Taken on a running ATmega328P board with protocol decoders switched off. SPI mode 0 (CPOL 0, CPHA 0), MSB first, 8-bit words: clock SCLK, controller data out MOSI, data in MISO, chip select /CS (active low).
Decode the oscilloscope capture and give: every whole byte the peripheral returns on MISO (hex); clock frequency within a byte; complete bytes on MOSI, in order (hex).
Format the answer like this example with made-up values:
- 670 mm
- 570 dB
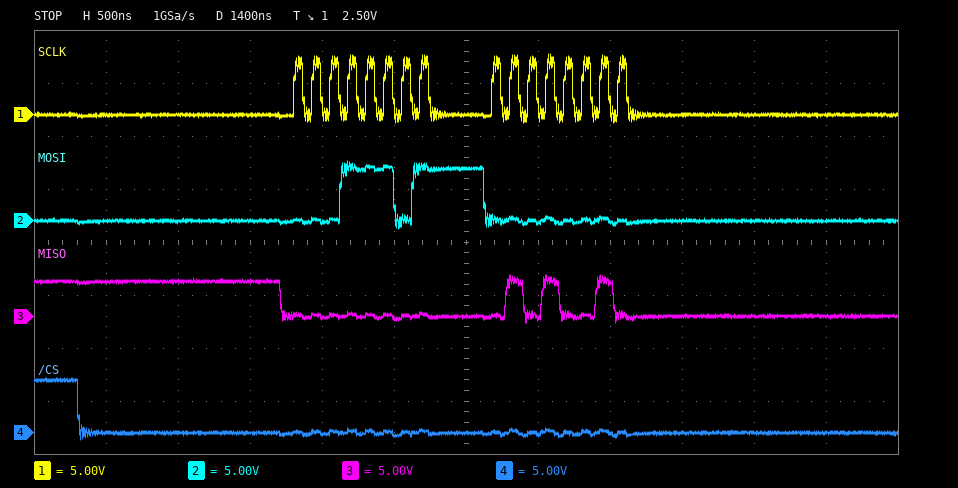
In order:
- 00 52
- 8 MHz
- 1D 00
